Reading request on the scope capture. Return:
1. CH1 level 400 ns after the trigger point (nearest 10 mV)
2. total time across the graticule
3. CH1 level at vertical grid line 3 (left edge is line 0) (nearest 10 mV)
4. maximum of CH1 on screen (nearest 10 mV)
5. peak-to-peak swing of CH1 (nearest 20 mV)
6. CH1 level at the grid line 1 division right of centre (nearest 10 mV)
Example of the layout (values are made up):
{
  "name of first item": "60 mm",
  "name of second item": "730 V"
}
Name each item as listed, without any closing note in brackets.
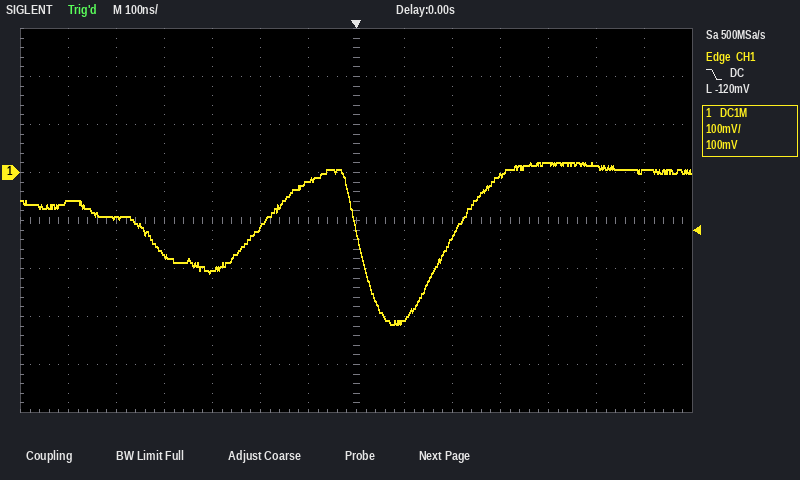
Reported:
{
  "CH1 level 400 ns after the trigger point": "20 mV",
  "total time across the graticule": "1.4 µs",
  "CH1 level at vertical grid line 3 (left edge is line 0)": "-170 mV",
  "maximum of CH1 on screen": "20 mV",
  "peak-to-peak swing of CH1": "340 mV",
  "CH1 level at the grid line 1 division right of centre": "-310 mV"
}
